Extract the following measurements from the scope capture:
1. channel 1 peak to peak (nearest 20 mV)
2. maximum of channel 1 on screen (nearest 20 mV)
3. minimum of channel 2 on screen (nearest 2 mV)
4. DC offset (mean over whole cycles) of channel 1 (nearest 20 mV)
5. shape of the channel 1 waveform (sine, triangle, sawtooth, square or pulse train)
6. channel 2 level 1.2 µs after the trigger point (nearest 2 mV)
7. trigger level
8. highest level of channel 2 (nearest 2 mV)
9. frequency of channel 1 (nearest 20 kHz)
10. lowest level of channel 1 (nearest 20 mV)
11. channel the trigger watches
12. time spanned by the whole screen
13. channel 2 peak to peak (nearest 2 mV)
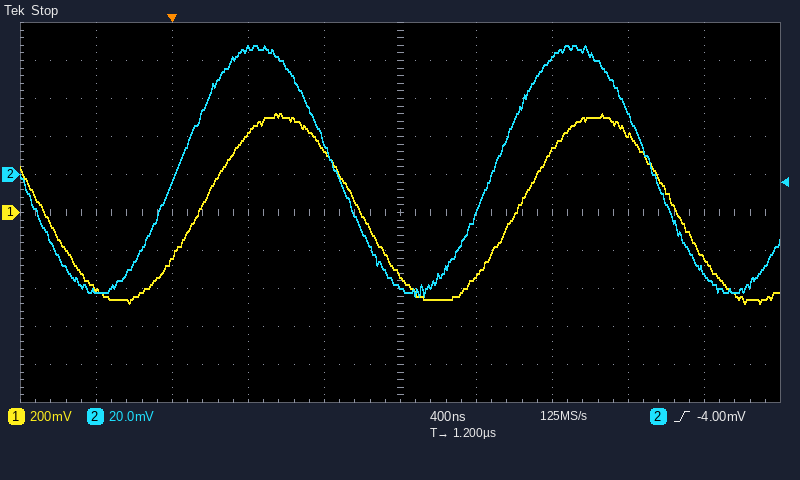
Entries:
1.00 V
520 mV
-64 mV
20 mV
sine
-60 mV
-4.00 mV
68 mV
600 kHz
-480 mV
channel 2
4 µs
132 mV
